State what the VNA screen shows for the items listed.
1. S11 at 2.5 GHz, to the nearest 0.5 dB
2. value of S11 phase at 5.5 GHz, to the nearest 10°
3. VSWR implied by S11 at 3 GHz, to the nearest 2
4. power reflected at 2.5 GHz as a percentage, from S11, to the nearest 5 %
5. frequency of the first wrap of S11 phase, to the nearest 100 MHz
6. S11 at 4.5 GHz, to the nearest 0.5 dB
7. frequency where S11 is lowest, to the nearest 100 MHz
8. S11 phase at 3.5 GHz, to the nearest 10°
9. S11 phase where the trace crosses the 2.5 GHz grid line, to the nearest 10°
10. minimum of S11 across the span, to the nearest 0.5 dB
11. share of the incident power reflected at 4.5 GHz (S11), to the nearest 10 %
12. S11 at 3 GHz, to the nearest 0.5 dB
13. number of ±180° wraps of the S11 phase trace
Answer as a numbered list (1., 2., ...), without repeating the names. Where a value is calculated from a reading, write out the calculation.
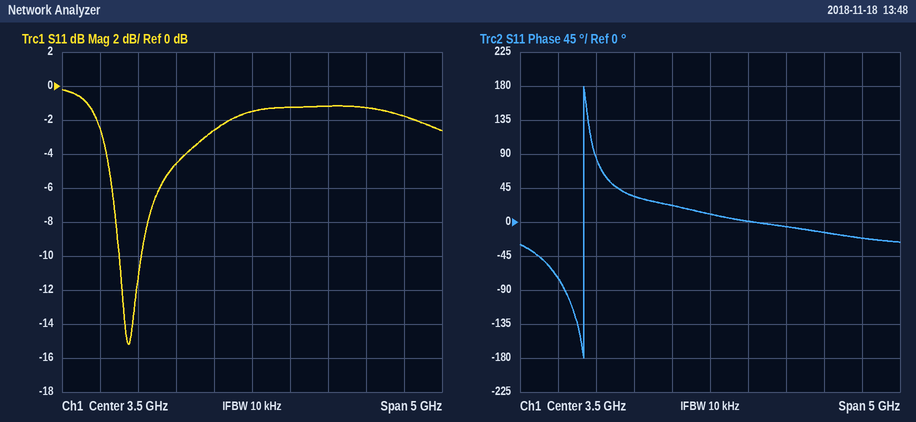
1. -4.5 dB
2. -20°
3. |Γ| = 10^(-2.5/20) = 0.7499; VSWR = (1 + 0.7499)/(1 − 0.7499) ≈ 7.00, so 6 to the nearest 2
4. 10^(-4.5/10) ≈ 35 %
5. 1.8 GHz
6. -1.0 dB
7. 1.9 GHz
8. 10°
9. 30°
10. -15.0 dB
11. 10^(-1/10) ≈ 79.4 %, so 80 % to the nearest 10 %
12. -2.5 dB
13. 1
